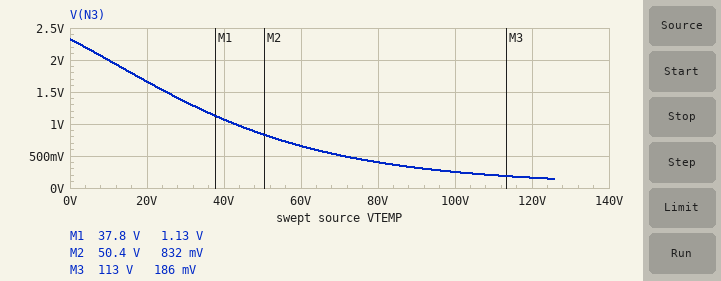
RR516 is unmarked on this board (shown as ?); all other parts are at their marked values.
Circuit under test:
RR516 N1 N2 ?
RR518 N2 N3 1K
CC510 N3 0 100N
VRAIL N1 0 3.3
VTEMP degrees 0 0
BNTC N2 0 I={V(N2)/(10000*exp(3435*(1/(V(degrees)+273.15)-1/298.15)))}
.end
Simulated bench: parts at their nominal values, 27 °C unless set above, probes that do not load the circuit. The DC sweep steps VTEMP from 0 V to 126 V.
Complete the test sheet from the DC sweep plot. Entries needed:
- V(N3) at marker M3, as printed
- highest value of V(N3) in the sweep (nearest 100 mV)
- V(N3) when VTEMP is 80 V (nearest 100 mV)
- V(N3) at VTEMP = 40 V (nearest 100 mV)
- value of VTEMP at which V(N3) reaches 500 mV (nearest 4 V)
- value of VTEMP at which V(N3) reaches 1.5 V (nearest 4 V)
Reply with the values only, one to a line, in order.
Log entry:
186 mV
2.3 V
400 mV
1.1 V
72 V
24 V
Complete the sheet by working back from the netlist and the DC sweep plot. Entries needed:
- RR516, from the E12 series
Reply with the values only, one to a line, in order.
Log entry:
12 kΩ
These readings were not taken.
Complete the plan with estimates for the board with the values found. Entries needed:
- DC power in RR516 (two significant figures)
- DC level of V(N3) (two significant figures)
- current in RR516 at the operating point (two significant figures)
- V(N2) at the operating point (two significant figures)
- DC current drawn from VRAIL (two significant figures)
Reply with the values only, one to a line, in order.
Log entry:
79 µW
2.3 V
81 µA
2.3 V
81 µA
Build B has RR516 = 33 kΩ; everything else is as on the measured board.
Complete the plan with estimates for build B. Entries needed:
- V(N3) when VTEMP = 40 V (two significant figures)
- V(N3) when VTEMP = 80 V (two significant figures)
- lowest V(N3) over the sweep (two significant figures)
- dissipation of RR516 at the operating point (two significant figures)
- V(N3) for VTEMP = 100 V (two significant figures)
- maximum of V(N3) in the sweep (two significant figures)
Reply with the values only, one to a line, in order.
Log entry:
490 mV
160 mV
53 mV
94 µW
96 mV
1.5 V
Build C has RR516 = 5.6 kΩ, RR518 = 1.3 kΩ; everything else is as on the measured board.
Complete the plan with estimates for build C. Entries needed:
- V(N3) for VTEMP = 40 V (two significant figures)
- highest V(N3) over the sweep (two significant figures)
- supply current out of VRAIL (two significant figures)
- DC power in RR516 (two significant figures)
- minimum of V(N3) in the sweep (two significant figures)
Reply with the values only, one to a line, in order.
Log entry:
1.7 V
2.8 V
96 µA
52 µW
290 mV
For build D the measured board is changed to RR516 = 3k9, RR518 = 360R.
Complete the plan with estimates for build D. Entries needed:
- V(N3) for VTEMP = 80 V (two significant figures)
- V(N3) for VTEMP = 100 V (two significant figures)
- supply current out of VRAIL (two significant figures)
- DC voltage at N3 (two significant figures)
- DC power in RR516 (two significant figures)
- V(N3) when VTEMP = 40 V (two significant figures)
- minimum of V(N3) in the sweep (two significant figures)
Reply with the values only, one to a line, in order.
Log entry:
990 mV
670 mV
100 µA
2.9 V
40 µW
2.0 V
400 mV
